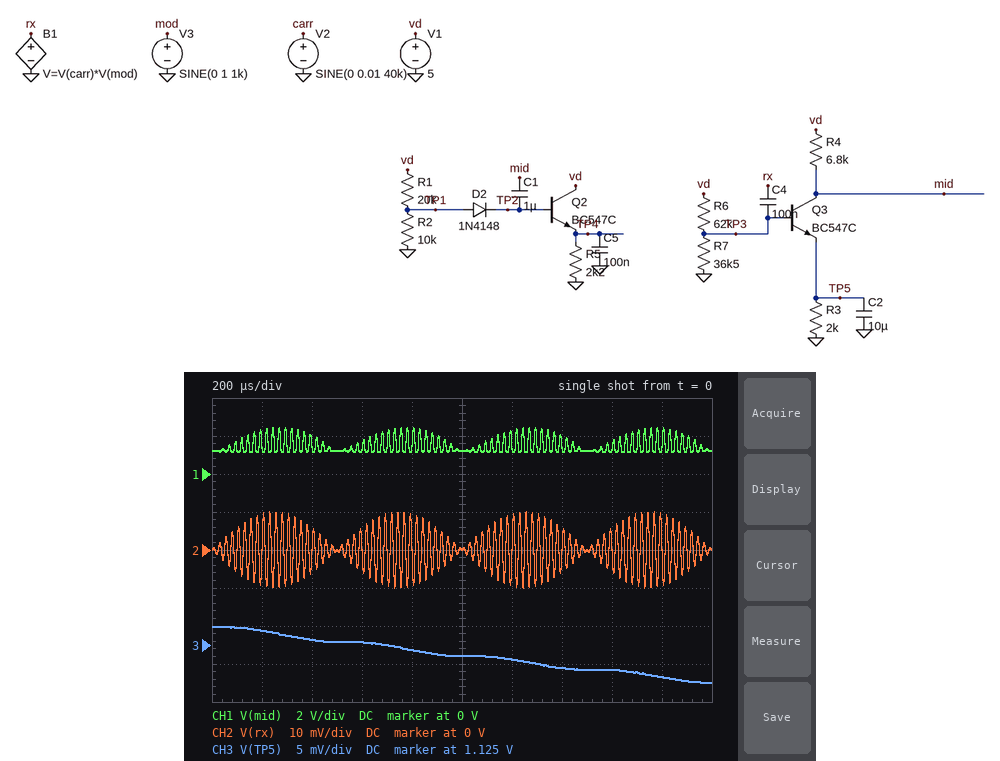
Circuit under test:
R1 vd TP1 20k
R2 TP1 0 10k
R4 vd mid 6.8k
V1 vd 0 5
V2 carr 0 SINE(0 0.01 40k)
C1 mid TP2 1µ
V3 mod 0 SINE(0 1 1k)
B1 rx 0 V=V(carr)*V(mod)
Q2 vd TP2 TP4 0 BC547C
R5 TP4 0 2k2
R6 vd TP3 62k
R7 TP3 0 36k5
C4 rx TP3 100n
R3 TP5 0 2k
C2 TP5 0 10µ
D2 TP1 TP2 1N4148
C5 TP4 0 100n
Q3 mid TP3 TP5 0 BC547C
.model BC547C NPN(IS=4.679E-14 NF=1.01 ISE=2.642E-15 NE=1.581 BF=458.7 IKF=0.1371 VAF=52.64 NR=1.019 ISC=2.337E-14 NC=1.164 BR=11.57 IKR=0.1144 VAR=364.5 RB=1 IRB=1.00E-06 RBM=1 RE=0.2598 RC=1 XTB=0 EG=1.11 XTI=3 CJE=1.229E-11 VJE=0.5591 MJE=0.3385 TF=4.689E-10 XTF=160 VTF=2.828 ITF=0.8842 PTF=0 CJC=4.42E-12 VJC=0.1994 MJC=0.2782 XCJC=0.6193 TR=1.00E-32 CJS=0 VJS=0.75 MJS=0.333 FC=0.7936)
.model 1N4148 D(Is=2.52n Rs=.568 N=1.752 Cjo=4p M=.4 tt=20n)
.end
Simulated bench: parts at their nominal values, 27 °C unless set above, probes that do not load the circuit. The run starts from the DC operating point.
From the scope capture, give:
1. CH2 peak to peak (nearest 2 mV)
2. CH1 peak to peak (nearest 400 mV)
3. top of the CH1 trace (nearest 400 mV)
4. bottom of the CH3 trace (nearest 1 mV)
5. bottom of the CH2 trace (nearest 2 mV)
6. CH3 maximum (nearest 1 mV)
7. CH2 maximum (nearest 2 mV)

20 mV
1.2 V
2.4 V
1.120 V
-10 mV
1.127 V
10 mV
